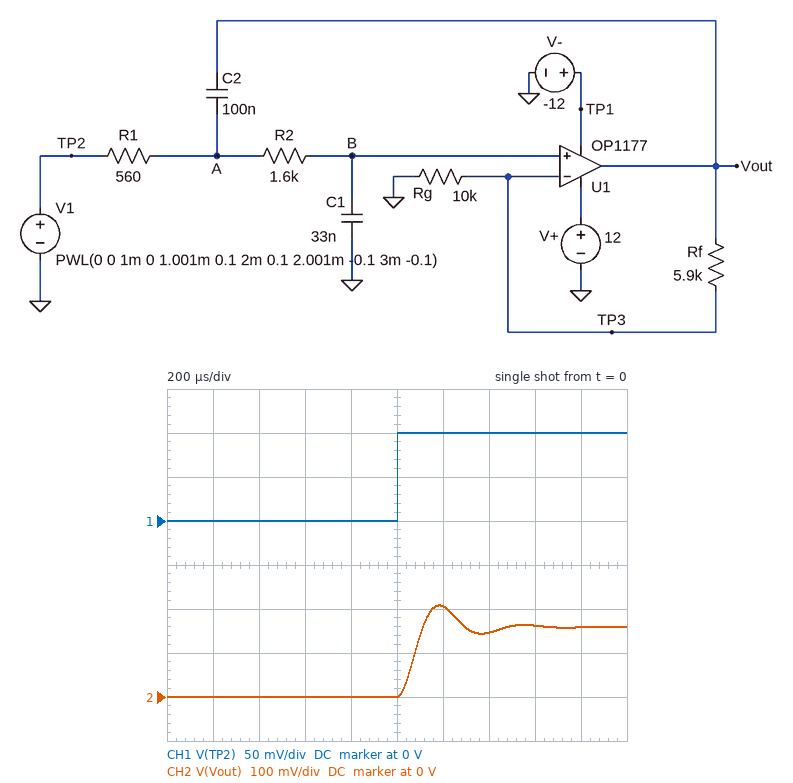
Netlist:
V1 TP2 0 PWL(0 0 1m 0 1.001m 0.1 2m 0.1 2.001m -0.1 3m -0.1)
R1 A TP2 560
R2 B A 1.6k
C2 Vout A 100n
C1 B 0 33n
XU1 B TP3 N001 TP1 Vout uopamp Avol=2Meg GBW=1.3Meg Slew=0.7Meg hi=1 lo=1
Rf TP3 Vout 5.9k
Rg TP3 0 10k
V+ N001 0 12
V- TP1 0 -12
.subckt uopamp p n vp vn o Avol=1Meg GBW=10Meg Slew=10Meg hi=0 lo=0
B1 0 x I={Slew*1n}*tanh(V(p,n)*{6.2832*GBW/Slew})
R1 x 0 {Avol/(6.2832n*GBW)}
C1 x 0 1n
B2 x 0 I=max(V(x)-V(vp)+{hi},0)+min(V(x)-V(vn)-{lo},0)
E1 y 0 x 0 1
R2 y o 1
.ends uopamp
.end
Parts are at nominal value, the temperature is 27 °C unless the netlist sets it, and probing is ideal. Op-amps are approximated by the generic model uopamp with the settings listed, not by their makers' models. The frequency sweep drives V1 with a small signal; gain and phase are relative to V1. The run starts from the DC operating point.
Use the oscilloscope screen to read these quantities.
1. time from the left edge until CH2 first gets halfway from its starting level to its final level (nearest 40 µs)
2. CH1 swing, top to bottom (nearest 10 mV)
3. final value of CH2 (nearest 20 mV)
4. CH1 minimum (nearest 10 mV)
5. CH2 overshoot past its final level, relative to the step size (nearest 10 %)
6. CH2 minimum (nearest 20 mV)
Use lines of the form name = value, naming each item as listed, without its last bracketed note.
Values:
time from the left edge until CH2 first gets halfway from its starting level to its final level = 1.08 ms
CH1 swing, top to bottom = 100 mV
final value of CH2 = 160 mV
CH1 minimum = 0 V
CH2 overshoot past its final level, relative to the step size = 30 %
CH2 minimum = 0 V
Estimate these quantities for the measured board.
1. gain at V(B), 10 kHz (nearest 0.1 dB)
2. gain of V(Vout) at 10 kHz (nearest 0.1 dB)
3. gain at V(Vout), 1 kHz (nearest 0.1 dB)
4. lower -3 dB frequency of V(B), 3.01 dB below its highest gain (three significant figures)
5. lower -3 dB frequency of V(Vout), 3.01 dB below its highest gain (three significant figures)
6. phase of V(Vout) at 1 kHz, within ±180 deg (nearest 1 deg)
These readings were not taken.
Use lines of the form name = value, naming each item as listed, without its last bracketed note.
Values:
gain at V(B), 10 kHz = -20.8 dB
gain of V(Vout) at 10 kHz = -16.8 dB
gain at V(Vout), 1 kHz = 4.8 dB
lower -3 dB frequency of V(B), 3.01 dB below its highest gain = 911 Hz
lower -3 dB frequency of V(Vout), 3.01 dB below its highest gain = 911 Hz
phase of V(Vout) at 1 kHz, within ±180 deg = -15 deg
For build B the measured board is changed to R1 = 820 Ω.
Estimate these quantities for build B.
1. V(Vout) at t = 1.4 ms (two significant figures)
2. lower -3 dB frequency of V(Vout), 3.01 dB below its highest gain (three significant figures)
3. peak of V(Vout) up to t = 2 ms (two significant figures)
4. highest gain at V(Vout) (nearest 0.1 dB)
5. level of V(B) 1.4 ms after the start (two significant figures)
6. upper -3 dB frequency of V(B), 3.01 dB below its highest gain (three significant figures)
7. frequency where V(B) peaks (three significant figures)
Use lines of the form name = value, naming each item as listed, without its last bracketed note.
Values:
V(Vout) at t = 1.4 ms = 130 mV
lower -3 dB frequency of V(Vout), 3.01 dB below its highest gain = 1.57 kHz
peak of V(Vout) up to t = 2 ms = 230 mV
highest gain at V(Vout) = 10.7 dB
level of V(B) 1.4 ms after the start = 81 mV
upper -3 dB frequency of V(B), 3.01 dB below its highest gain = 2.80 kHz
frequency where V(B) peaks = 2.27 kHz
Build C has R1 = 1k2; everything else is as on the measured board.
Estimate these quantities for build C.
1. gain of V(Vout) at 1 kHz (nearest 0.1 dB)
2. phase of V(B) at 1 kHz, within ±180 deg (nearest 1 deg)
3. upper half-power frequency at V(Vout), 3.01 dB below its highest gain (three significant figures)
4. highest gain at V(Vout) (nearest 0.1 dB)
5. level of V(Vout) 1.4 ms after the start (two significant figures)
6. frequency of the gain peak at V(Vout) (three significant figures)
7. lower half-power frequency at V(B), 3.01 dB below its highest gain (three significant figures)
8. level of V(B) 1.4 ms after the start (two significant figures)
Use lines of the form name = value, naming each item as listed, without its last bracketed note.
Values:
gain of V(Vout) at 1 kHz = 6.4 dB
phase of V(B) at 1 kHz, within ±180 deg = -10 deg
upper half-power frequency at V(Vout), 3.01 dB below its highest gain = 2.21 kHz
highest gain at V(Vout) = 15.5 dB
level of V(Vout) 1.4 ms after the start = 150 mV
frequency of the gain peak at V(Vout) = 1.96 kHz
lower half-power frequency at V(B), 3.01 dB below its highest gain = 1.66 kHz
level of V(B) 1.4 ms after the start = 94 mV
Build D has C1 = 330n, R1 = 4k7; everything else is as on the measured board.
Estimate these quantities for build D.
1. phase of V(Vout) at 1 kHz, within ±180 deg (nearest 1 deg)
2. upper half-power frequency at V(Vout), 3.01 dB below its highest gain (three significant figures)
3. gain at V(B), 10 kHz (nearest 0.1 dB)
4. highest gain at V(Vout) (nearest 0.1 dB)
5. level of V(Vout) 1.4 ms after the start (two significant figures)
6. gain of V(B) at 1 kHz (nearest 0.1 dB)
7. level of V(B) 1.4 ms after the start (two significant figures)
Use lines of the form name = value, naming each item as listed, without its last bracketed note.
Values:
phase of V(Vout) at 1 kHz, within ±180 deg = -128 deg
upper half-power frequency at V(Vout), 3.01 dB below its highest gain = 95.6 Hz
gain at V(B), 10 kHz = -59.9 dB
highest gain at V(Vout) = 4.0 dB
level of V(Vout) 1.4 ms after the start = 23 mV
gain of V(B) at 1 kHz = -23.1 dB
level of V(B) 1.4 ms after the start = 14 mV
